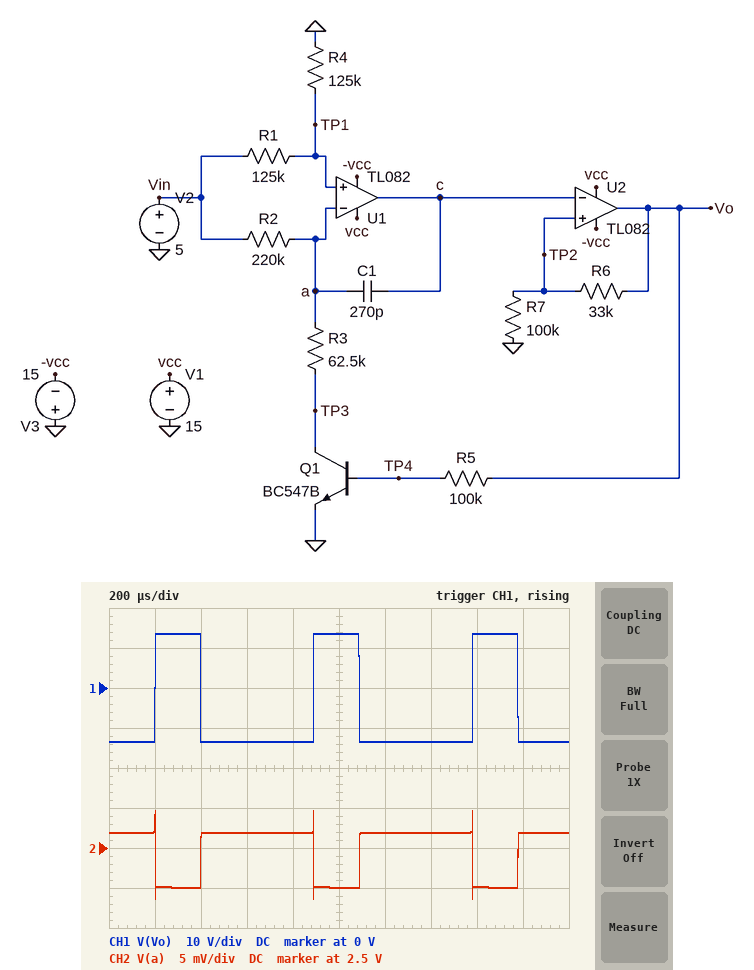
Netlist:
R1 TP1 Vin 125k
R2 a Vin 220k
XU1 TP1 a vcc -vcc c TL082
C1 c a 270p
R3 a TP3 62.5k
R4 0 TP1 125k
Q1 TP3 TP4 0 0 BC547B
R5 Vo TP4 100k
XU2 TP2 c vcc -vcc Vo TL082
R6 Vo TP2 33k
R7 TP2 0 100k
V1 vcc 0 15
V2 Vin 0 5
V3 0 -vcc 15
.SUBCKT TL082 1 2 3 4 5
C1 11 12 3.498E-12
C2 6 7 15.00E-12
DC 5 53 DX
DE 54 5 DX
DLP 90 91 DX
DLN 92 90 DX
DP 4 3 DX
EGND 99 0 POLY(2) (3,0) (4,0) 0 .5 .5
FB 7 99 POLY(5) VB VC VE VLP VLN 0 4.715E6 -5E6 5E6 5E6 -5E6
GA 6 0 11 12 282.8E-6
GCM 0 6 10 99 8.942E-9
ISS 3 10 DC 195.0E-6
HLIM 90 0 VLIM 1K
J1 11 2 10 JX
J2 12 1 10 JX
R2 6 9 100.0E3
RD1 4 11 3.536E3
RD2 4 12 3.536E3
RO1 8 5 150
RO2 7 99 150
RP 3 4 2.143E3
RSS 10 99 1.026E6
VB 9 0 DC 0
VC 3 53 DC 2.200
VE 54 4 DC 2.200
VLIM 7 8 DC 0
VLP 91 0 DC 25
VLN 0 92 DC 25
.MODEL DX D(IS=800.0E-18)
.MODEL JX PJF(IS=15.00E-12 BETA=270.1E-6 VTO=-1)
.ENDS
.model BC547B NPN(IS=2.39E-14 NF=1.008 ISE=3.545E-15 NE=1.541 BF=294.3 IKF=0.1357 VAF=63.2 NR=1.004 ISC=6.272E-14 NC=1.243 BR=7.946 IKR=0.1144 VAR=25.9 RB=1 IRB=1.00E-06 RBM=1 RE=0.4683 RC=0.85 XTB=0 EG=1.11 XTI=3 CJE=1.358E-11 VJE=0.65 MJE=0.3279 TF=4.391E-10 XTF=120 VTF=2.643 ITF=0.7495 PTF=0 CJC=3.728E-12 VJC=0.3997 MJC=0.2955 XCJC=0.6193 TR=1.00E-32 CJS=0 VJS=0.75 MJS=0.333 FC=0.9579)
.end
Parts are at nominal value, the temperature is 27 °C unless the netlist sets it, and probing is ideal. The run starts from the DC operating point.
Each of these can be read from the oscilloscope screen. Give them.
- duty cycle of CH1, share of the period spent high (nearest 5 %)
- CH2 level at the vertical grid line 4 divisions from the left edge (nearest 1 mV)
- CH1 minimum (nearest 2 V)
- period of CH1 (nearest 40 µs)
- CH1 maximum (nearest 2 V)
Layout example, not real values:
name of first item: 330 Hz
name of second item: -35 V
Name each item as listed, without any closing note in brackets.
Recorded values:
duty cycle of CH1, share of the period spent high: 30 %
CH2 level at the vertical grid line 4 divisions from the left edge: 2.502 V
CH1 minimum: -14 V
period of CH1: 680 µs
CH1 maximum: 14 V
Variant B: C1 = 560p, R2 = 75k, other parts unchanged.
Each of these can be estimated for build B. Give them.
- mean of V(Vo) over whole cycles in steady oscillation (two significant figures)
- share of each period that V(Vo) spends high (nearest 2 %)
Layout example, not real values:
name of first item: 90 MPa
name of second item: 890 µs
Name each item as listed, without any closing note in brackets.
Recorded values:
mean of V(Vo) over whole cycles in steady oscillation: 9.1 V
share of each period that V(Vo) spends high: 84 %
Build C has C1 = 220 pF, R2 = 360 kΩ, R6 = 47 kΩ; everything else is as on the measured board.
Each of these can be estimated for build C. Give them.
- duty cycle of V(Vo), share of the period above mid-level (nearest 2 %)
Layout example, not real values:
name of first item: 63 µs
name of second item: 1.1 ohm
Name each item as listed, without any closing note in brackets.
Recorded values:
duty cycle of V(Vo), share of the period above mid-level: 18 %
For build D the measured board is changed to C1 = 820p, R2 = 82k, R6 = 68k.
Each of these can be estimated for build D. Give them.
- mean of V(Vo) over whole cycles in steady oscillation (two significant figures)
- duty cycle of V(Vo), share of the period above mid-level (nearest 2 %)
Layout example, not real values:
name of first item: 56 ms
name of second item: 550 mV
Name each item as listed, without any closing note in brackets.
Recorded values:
mean of V(Vo) over whole cycles in steady oscillation: 7.1 V
duty cycle of V(Vo), share of the period above mid-level: 76 %
